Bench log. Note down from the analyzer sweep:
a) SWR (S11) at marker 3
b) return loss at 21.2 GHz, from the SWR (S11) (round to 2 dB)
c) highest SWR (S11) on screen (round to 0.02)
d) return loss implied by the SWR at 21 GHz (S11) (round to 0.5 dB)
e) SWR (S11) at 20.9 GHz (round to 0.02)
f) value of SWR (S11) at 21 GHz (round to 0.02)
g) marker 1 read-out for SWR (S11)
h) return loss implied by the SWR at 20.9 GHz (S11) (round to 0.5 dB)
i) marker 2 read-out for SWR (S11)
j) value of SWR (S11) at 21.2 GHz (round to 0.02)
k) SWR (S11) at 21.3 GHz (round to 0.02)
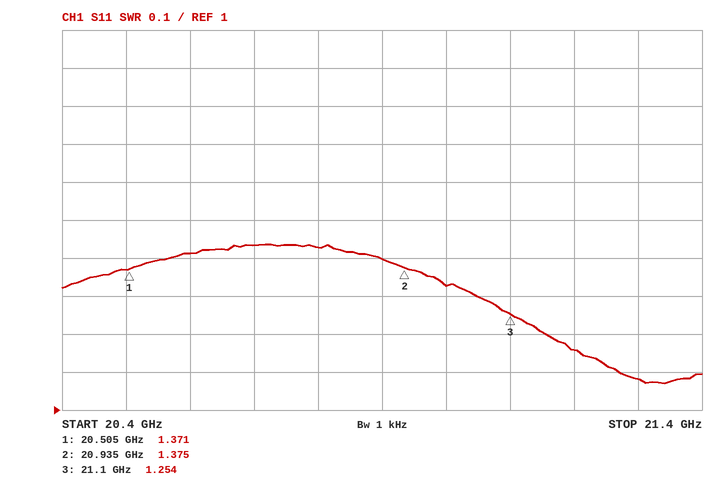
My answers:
1.254
22 dB
1.44
17.0 dB
1.40
1.32
1.371
15.5 dB
1.375
1.16
1.08
